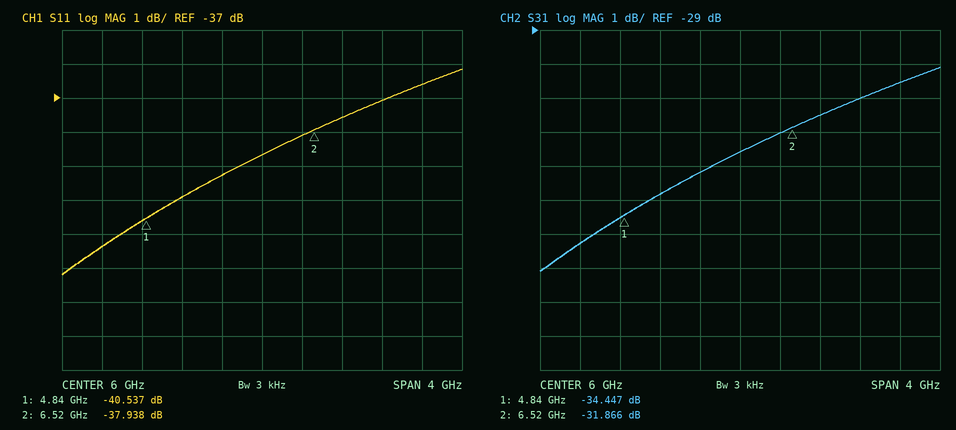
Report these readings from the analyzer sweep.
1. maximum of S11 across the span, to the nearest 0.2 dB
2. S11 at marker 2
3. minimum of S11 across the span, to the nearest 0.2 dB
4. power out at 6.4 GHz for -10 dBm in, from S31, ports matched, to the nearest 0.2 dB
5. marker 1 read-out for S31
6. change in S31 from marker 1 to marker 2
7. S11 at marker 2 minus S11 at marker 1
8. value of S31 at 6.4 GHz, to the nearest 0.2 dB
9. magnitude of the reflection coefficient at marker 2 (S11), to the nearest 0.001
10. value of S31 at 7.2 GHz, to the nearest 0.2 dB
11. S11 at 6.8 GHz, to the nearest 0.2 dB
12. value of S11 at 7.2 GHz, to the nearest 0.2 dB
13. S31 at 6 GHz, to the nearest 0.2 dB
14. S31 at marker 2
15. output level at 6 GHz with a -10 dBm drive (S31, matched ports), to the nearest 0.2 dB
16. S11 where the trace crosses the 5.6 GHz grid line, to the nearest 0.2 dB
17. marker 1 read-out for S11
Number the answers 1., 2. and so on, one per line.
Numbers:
1. -36.2 dB
2. -37.938 dB
3. -42.2 dB
4. -42.0 dBm
5. -34.447 dB
6. 2.581 dB
7. 2.599 dB
8. -32.0 dB
9. 0.013
10. -31.0 dB
11. -37.6 dB
12. -37.0 dB
13. -32.6 dB
14. -31.866 dB
15. -42.6 dBm
16. -39.2 dB
17. -40.537 dB
